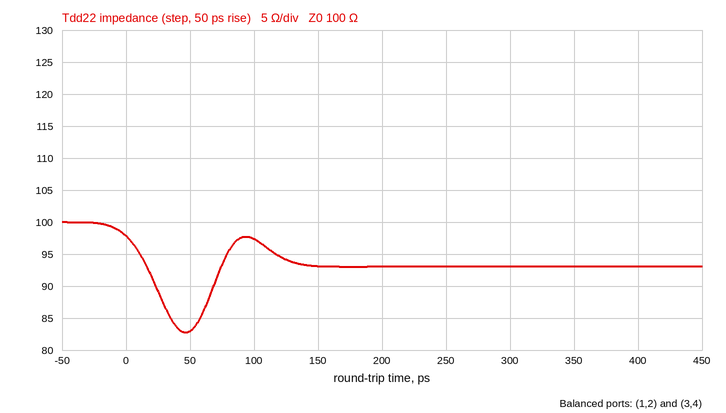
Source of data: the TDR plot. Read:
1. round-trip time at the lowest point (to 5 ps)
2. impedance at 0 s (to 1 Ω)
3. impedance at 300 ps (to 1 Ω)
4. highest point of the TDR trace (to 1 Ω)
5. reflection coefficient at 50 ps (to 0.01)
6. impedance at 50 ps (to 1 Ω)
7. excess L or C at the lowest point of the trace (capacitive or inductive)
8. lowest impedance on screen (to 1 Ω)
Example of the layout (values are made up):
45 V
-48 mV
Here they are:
45 ps
98 Ω
93 Ω
100 Ω
-0.09
83 Ω
capacitive
83 Ω
